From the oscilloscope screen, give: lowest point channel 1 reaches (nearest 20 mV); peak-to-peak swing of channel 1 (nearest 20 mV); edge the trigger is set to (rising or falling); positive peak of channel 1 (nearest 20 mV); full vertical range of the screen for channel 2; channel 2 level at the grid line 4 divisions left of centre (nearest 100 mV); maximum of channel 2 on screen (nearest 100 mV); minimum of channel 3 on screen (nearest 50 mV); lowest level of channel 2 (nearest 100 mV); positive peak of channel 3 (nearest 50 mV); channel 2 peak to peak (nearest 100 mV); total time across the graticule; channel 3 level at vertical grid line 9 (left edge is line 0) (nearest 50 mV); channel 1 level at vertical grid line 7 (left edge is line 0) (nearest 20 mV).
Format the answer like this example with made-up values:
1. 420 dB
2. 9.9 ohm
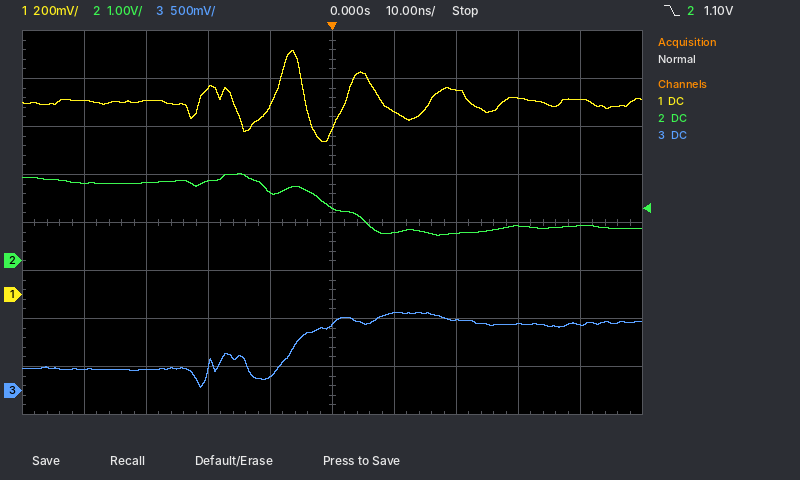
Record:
1. 640 mV
2. 380 mV
3. falling
4. 1.02 V
5. 8 V
6. 1.6 V
7. 1.8 V
8. 50 mV
9. 500 mV
10. 800 mV
11. 1.3 V
12. 100 ns
13. 700 mV
14. 860 mV
